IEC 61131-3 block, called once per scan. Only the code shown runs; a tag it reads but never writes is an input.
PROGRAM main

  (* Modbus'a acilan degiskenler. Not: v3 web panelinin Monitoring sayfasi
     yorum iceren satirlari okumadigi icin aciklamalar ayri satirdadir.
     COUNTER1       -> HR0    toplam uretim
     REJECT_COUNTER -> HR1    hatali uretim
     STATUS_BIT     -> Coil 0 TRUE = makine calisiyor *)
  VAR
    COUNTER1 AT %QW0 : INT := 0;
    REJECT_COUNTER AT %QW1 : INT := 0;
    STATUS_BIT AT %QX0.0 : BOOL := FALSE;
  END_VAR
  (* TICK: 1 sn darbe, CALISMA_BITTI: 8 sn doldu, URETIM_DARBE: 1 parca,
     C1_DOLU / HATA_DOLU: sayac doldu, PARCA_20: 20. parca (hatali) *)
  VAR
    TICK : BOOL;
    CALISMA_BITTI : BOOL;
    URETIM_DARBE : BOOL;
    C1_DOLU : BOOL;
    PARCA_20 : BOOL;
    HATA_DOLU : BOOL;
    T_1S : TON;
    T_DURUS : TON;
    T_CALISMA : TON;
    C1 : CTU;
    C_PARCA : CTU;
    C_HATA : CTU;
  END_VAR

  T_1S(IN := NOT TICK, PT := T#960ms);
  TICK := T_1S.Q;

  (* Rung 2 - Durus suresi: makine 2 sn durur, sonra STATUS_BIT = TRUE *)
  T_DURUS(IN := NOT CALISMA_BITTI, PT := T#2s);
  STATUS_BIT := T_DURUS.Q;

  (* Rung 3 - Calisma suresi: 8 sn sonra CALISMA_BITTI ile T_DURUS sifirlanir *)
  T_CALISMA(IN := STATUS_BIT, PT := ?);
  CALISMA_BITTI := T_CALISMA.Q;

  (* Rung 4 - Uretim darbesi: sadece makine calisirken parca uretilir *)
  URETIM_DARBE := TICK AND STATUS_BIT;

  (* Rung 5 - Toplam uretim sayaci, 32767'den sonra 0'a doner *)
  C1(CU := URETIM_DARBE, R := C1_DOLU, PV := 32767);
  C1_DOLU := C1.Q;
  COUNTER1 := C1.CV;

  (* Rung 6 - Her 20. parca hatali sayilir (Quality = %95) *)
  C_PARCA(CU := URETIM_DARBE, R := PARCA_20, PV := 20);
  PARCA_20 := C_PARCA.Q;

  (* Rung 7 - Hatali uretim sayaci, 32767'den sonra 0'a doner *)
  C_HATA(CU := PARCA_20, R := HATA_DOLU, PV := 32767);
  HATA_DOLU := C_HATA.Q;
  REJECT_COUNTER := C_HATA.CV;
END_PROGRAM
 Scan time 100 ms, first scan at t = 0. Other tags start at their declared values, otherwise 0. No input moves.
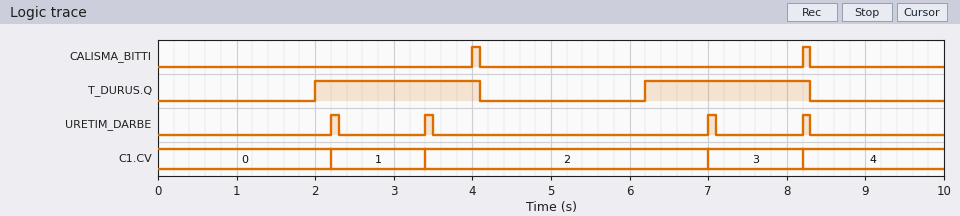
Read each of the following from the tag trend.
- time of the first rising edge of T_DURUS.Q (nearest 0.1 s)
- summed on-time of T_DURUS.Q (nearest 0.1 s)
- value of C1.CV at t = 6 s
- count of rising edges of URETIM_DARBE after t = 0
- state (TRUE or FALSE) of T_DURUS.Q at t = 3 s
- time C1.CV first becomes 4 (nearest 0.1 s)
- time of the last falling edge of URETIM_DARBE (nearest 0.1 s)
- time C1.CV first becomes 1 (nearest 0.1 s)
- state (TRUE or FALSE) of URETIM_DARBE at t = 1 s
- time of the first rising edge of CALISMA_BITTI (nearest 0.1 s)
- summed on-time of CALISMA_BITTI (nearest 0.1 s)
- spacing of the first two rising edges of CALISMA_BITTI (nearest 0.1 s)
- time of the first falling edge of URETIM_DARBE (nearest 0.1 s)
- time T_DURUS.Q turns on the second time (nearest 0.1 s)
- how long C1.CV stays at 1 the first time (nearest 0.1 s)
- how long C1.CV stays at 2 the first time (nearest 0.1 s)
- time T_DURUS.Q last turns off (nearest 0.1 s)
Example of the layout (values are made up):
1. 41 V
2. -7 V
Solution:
1. 2.0 s
2. 4.2 s
3. 2
4. 4
5. TRUE
6. 8.2 s
7. 8.3 s
8. 2.2 s
9. FALSE
10. 4.0 s
11. 0.2 s
12. 4.2 s
13. 2.3 s
14. 6.2 s
15. 1.2 s
16. 3.6 s
17. 8.3 s
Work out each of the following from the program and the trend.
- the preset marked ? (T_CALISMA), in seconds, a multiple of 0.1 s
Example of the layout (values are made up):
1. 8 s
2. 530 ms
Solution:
1. 2.0 s
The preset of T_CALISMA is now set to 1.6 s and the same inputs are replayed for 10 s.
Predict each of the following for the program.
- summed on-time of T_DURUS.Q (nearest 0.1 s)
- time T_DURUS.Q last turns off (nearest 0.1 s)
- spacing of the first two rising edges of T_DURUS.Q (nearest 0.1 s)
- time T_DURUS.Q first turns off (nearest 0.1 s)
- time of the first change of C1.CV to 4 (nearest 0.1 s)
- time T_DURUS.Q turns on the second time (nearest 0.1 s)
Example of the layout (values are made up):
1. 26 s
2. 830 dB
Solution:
1. 3.8 s
2. 7.5 s
3. 3.8 s
4. 3.7 s
5. 7.0 s
6. 5.8 s
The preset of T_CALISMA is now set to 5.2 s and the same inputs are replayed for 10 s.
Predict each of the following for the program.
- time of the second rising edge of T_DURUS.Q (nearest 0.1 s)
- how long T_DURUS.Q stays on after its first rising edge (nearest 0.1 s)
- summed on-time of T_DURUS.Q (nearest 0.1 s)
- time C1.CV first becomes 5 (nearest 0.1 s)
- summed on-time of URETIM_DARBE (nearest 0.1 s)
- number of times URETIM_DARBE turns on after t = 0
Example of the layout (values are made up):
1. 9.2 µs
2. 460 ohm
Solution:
1. 9.4 s
2. 5.3 s
3. 5.9 s
4. 7.0 s
5. 0.6 s
6. 6
